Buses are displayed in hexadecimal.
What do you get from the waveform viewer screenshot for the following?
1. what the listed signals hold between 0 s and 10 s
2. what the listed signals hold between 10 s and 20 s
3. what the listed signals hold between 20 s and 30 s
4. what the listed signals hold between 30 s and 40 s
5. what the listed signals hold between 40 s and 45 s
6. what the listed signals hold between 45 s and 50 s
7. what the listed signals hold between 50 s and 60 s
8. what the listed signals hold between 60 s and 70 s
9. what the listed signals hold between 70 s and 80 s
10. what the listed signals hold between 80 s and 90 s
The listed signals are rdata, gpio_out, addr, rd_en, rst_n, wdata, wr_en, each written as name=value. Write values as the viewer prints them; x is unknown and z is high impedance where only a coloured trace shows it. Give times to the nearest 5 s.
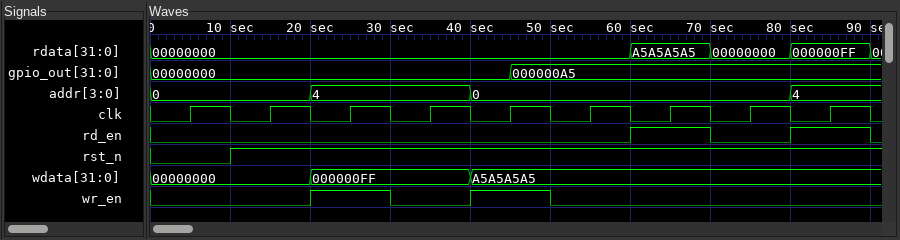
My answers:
rdata=00000000, gpio_out=00000000, addr=0, rd_en=0, rst_n=0, wdata=00000000, wr_en=0
rdata=00000000, gpio_out=00000000, addr=0, rd_en=0, rst_n=1, wdata=00000000, wr_en=0
rdata=00000000, gpio_out=00000000, addr=4, rd_en=0, rst_n=1, wdata=000000FF, wr_en=1
rdata=00000000, gpio_out=00000000, addr=4, rd_en=0, rst_n=1, wdata=000000FF, wr_en=0
rdata=00000000, gpio_out=00000000, addr=0, rd_en=0, rst_n=1, wdata=A5A5A5A5, wr_en=1
rdata=00000000, gpio_out=000000A5, addr=0, rd_en=0, rst_n=1, wdata=A5A5A5A5, wr_en=1
rdata=00000000, gpio_out=000000A5, addr=0, rd_en=0, rst_n=1, wdata=A5A5A5A5, wr_en=0
rdata=A5A5A5A5, gpio_out=000000A5, addr=0, rd_en=1, rst_n=1, wdata=A5A5A5A5, wr_en=0
rdata=00000000, gpio_out=000000A5, addr=0, rd_en=0, rst_n=1, wdata=A5A5A5A5, wr_en=0
rdata=000000FF, gpio_out=000000A5, addr=4, rd_en=1, rst_n=1, wdata=A5A5A5A5, wr_en=0
